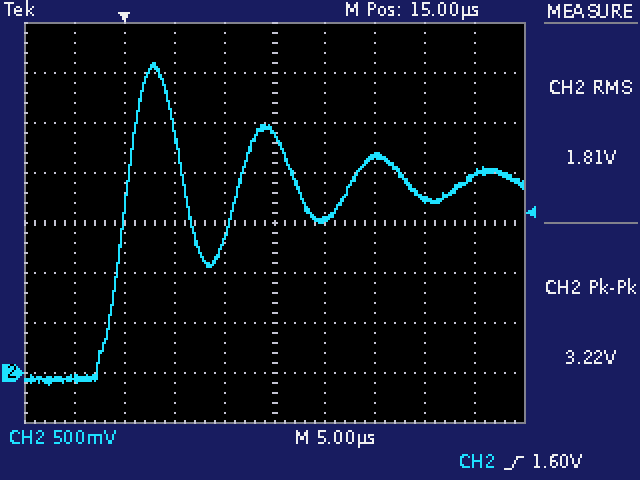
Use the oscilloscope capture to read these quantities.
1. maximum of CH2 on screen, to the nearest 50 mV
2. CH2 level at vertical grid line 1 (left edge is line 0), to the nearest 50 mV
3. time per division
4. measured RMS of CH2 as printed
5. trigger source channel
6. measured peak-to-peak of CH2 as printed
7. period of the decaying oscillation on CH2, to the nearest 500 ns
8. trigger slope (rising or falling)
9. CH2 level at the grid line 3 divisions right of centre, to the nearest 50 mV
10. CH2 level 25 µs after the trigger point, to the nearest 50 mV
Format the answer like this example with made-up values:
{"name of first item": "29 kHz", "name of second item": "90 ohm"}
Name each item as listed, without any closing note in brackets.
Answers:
{"maximum of CH2 on screen, to the nearest 50 mV": "3.10 V", "CH2 level at vertical grid line 1 (left edge is line 0), to the nearest 50 mV": "-50 mV", "time per division": "5 µs", "measured RMS of CH2 as printed": "1.81 V", "trigger source channel": "CH2", "measured peak-to-peak of CH2 as printed": "3.22 V", "period of the decaying oscillation on CH2, to the nearest 500 ns": "11.5 µs", "trigger slope": "rising", "CH2 level at the grid line 3 divisions right of centre, to the nearest 50 mV": "1.75 V", "CH2 level 25 µs after the trigger point, to the nearest 50 mV": "2.15 V"}
